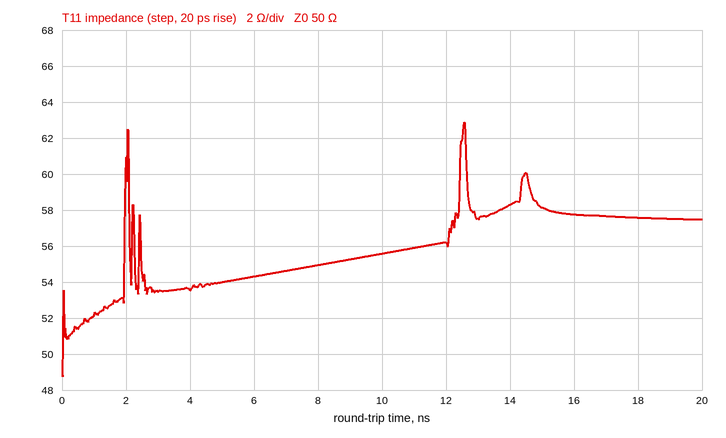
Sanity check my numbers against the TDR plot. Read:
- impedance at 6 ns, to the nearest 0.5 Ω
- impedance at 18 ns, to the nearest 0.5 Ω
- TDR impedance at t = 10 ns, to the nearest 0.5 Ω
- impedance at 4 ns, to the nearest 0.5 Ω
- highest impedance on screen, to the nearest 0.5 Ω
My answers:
54.5 Ω
57.5 Ω
55.5 Ω
53.5 Ω
63.0 Ω
